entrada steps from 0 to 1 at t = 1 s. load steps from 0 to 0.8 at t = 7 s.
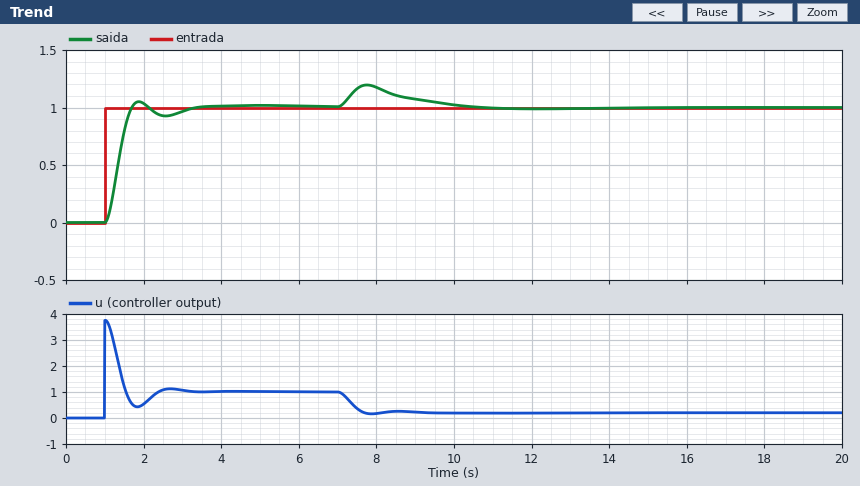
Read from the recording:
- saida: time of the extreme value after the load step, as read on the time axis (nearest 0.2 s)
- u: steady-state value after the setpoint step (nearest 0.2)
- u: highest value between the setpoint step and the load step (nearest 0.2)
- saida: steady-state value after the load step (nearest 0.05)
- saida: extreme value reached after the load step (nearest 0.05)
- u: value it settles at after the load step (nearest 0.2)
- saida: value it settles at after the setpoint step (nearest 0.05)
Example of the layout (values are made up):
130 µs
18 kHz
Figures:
7.8 s
1.0
3.8
1.00
1.20
0.2
1.00
